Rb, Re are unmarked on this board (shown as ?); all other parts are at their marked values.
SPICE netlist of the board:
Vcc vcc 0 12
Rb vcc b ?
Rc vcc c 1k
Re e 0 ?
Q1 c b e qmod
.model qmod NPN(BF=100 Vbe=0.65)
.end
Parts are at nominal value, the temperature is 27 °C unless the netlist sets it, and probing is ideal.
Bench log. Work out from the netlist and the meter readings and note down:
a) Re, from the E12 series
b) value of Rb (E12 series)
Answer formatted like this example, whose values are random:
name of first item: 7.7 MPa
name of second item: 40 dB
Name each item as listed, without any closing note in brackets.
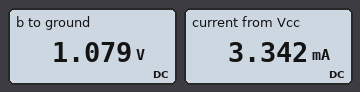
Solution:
Re, from the E12 series: 82 Ω
value of Rb: 330 kΩ
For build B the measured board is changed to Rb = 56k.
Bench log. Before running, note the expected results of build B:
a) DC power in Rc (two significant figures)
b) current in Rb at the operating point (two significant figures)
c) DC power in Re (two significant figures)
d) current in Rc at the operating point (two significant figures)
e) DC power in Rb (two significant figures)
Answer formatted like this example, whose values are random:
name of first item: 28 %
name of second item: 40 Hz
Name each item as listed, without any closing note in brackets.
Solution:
DC power in Rc: 120 mW
current in Rb at the operating point: 180 µA
DC power in Re: 10 mW
current in Rc at the operating point: 11 mA
DC power in Rb: 1.9 mW
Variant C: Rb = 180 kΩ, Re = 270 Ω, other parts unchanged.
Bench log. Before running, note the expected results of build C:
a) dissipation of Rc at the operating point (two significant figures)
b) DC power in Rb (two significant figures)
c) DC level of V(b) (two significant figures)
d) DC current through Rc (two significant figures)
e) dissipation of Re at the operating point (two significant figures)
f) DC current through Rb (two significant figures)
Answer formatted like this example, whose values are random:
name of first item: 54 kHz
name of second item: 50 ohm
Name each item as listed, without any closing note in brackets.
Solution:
dissipation of Rc at the operating point: 29 mW
DC power in Rb: 520 µW
DC level of V(b): 2.3 V
DC current through Rc: 5.4 mA
dissipation of Re at the operating point: 8.0 mW
DC current through Rb: 54 µA
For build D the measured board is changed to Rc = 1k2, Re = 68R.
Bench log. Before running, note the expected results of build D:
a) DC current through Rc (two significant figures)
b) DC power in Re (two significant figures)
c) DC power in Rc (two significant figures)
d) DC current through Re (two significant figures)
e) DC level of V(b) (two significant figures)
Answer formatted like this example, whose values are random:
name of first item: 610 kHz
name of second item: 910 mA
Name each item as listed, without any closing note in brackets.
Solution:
DC current through Rc: 3.3 mA
DC power in Re: 770 µW
DC power in Rc: 13 mW
DC current through Re: 3.4 mA
DC level of V(b): 1.0 V
